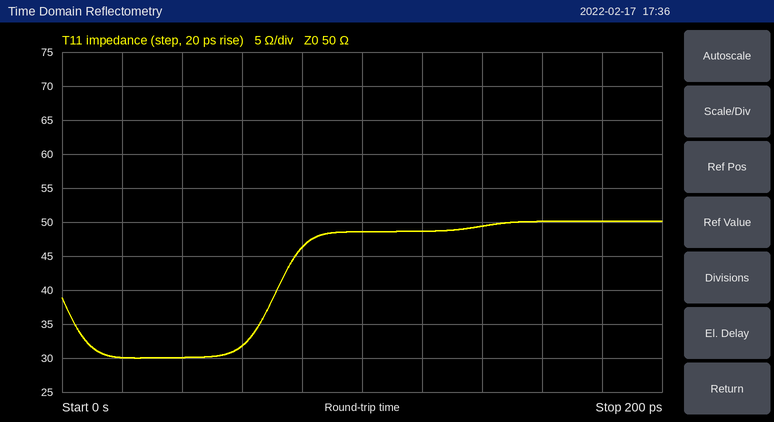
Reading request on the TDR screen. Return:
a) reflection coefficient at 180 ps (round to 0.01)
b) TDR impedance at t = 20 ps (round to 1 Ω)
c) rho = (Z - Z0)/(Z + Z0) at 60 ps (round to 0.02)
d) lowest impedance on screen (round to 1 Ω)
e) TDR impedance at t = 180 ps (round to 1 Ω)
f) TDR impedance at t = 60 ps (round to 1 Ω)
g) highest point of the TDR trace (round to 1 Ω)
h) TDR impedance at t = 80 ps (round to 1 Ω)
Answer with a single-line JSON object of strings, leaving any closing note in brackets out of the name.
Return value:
{"reflection coefficient at 180 ps": "0.00", "TDR impedance at t = 20 ps": "30 Ω", "rho = (Z - Z0)/(Z + Z0) at 60 ps": "-0.22", "lowest impedance on screen": "30 Ω", "TDR impedance at t = 180 ps": "50 Ω", "TDR impedance at t = 60 ps": "32 Ω", "highest point of the TDR trace": "50 Ω", "TDR impedance at t = 80 ps": "46 Ω"}
